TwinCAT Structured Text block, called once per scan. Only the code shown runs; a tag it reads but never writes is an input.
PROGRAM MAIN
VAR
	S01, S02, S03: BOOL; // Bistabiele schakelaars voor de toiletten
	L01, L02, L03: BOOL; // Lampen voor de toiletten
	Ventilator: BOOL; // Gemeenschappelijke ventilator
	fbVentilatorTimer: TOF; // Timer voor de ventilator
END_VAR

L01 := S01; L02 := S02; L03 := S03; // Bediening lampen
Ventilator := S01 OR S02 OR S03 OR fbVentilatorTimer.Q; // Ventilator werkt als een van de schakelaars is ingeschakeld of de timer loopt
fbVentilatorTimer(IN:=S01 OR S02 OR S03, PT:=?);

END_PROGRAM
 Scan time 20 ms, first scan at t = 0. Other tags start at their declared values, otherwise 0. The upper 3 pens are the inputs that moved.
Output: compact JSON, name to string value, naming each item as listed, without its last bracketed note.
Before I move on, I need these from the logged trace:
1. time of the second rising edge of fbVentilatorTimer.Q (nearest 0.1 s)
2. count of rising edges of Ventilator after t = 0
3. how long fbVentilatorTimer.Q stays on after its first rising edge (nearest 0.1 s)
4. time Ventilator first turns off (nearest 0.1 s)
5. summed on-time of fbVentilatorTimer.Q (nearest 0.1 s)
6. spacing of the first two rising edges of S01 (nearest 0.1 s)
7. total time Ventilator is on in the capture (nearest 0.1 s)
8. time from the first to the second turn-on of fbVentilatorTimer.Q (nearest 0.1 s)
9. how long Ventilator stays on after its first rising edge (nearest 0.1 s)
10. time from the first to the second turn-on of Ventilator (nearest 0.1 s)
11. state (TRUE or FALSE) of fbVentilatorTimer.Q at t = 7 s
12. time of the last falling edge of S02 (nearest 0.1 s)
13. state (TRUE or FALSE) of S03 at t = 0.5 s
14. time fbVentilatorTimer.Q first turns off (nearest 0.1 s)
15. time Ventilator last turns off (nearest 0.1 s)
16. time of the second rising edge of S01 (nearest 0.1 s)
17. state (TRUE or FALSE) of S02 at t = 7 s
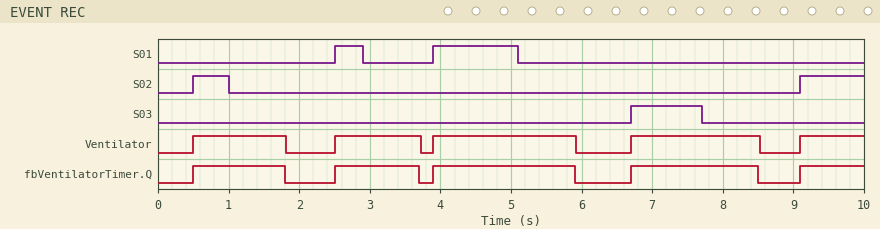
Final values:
{"time of the second rising edge of fbVentilatorTimer.Q": "2.5 s", "count of rising edges of Ventilator after t = 0": "5", "how long fbVentilatorTimer.Q stays on after its first rising edge": "1.3 s", "time Ventilator first turns off": "1.8 s", "summed on-time of fbVentilatorTimer.Q": "7.2 s", "spacing of the first two rising edges of S01": "1.4 s", "total time Ventilator is on in the capture": "7.3 s", "time from the first to the second turn-on of fbVentilatorTimer.Q": "2.0 s", "how long Ventilator stays on after its first rising edge": "1.3 s", "time from the first to the second turn-on of Ventilator": "2.0 s", "state (TRUE or FALSE) of fbVentilatorTimer.Q at t = 7 s": "TRUE", "time of the last falling edge of S02": "1.0 s", "state (TRUE or FALSE) of S03 at t = 0.5 s": "FALSE", "time fbVentilatorTimer.Q first turns off": "1.8 s", "time Ventilator last turns off": "8.5 s", "time of the second rising edge of S01": "3.9 s", "state (TRUE or FALSE) of S02 at t = 7 s": "FALSE"}
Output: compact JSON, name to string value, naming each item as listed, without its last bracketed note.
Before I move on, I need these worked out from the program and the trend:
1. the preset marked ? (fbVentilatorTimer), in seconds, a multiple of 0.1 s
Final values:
{"the preset marked ? (fbVentilatorTimer), in seconds, a multiple of 0.1 s": "0.8 s"}
